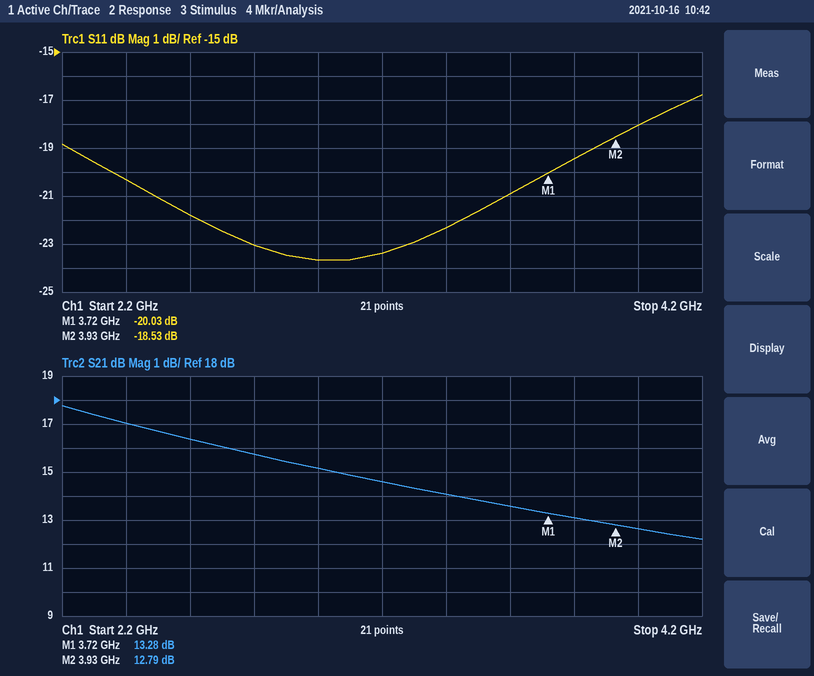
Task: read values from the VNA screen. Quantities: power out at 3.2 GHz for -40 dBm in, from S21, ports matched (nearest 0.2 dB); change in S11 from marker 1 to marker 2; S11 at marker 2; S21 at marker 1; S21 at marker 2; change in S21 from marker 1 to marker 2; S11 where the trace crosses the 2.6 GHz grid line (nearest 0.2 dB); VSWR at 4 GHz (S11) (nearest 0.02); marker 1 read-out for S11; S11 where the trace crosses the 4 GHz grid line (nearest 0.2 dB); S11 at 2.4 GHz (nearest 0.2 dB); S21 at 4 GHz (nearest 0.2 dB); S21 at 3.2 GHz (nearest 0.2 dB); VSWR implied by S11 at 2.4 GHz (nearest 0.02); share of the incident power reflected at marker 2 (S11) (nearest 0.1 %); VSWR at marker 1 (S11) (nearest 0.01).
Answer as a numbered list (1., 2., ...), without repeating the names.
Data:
1. -25.4 dBm
2. 1.50 dB
3. -18.53 dB
4. 13.28 dB
5. 12.79 dB
6. -0.49 dB
7. -21.8 dB
8. 1.28
9. -20.03 dB
10. -18.0 dB
11. -20.4 dB
12. 12.6 dB
13. 14.6 dB
14. 1.22
15. 1.4 %
16. 1.22
